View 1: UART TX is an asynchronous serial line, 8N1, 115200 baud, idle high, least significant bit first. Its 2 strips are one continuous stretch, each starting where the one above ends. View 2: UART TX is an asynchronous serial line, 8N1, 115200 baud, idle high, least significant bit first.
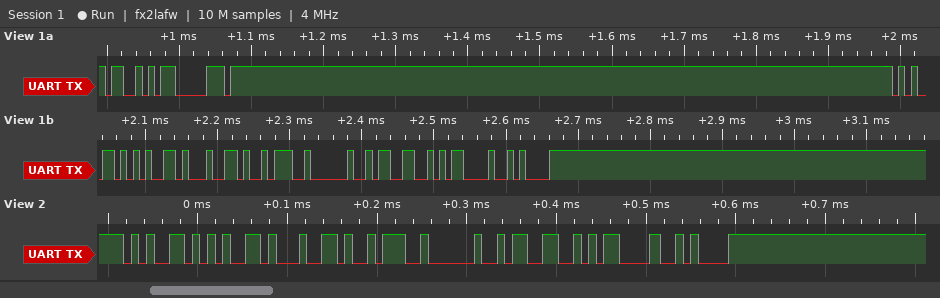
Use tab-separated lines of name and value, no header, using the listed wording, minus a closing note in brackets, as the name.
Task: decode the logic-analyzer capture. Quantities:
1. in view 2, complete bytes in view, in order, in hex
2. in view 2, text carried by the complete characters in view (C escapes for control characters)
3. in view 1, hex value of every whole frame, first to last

in view 2, complete bytes in view, in order, in hex	65 65 64 3A 20 33 0D 0A
in view 2, text carried by the complete characters in view	"eed: 3\r\n"
in view 1, hex value of every whole frame, first to last	53 70 65 65 64 3A 20 33 0D 0A
